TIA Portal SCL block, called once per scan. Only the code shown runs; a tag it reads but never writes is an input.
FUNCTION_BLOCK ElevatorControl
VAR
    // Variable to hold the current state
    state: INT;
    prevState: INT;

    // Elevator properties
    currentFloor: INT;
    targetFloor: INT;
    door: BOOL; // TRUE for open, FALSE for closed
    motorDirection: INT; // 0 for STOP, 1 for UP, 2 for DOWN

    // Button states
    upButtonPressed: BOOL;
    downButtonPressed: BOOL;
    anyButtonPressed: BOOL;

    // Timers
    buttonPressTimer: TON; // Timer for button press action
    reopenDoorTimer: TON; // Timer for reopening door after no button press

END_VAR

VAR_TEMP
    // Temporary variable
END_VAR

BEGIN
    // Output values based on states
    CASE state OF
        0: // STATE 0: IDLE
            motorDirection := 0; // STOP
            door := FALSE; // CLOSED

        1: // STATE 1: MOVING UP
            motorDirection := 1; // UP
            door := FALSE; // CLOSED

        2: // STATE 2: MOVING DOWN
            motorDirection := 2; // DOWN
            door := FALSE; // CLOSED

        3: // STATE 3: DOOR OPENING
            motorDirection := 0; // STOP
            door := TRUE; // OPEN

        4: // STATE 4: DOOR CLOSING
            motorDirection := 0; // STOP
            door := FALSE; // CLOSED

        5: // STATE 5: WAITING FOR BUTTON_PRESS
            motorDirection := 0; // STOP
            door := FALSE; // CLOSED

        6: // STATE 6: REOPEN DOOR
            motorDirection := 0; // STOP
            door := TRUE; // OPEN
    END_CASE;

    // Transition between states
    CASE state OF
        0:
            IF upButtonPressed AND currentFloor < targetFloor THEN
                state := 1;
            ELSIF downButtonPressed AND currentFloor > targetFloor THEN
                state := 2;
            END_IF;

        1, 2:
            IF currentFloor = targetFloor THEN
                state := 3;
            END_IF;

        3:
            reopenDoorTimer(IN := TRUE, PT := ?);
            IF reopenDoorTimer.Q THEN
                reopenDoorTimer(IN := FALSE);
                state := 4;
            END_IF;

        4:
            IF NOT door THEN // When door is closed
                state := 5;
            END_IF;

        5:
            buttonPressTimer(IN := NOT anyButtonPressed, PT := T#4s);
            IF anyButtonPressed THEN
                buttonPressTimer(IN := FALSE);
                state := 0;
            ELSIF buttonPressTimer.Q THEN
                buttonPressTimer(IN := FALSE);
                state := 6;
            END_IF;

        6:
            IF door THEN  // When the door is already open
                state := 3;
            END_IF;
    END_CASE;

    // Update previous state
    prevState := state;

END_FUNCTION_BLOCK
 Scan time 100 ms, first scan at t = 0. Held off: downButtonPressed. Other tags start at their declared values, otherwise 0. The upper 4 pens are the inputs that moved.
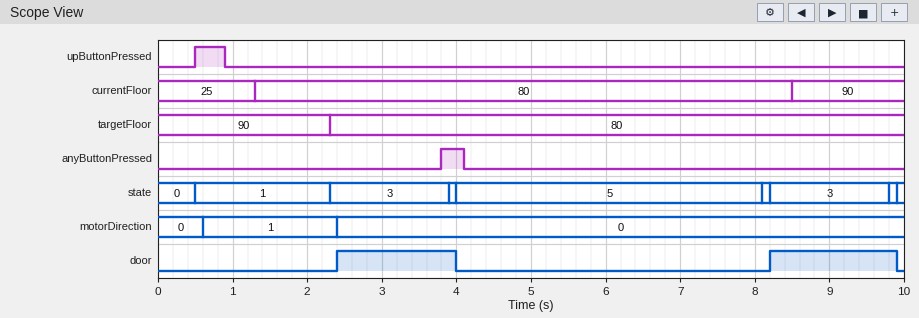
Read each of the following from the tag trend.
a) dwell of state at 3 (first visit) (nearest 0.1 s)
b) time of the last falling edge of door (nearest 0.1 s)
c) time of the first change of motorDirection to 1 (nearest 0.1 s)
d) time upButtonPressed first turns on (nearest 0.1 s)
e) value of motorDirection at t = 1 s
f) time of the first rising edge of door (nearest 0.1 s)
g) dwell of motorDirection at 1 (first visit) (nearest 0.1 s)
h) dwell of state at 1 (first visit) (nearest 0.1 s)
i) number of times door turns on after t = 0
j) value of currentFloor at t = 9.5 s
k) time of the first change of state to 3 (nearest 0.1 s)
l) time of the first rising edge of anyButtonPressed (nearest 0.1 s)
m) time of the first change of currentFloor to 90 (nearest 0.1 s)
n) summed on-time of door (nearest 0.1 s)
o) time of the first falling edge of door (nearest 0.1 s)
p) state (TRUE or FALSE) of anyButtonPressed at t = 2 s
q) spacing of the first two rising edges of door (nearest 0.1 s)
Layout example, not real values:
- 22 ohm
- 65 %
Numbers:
- 1.6 s
- 9.9 s
- 0.6 s
- 0.5 s
- 1
- 2.4 s
- 1.8 s
- 1.8 s
- 2
- 90
- 2.3 s
- 3.8 s
- 8.5 s
- 3.3 s
- 4.0 s
- FALSE
- 5.8 s
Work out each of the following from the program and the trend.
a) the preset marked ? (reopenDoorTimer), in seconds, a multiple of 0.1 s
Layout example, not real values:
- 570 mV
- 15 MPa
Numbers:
- 1.5 s
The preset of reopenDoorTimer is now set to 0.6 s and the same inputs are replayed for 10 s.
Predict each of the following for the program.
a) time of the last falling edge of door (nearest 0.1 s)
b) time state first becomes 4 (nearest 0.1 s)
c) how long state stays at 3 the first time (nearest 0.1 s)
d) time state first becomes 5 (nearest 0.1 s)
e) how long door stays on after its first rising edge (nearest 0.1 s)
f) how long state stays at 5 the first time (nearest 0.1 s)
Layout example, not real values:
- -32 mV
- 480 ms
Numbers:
- 3.1 s
- 3.0 s
- 0.7 s
- 3.1 s
- 0.7 s
- 0.7 s
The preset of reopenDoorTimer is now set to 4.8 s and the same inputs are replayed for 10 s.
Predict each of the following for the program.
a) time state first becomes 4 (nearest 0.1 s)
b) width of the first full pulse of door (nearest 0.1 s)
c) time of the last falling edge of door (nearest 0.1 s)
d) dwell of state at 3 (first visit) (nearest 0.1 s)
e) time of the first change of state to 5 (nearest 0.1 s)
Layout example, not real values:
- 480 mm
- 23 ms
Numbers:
- 7.2 s
- 4.9 s
- 7.3 s
- 4.9 s
- 7.3 s
